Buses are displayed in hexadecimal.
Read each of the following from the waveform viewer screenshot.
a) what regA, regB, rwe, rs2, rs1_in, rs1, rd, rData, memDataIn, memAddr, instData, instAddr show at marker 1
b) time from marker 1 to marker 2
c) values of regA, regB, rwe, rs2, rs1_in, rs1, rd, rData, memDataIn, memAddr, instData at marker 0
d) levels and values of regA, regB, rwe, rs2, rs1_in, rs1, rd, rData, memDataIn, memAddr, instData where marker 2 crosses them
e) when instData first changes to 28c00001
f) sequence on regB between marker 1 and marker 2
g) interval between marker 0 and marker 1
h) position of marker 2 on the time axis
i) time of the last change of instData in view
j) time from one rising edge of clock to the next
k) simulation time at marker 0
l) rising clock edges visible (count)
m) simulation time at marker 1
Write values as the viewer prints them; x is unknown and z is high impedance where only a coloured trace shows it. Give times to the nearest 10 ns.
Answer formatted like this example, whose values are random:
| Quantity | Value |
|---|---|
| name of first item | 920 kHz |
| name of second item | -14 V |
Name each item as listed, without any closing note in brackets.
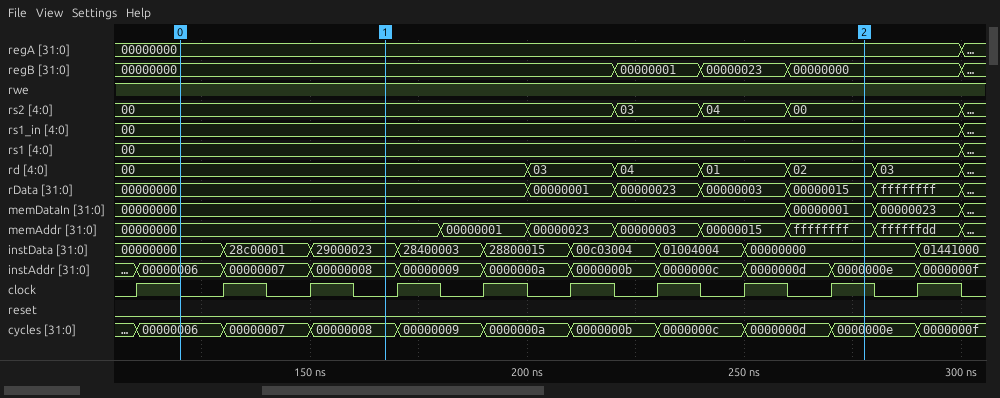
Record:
| Quantity | Value |
|---|---|
| what regA, regB, rwe, rs2, rs1_in, rs1, rd, rData, memDataIn, memAddr, instData, instAddr show at marker 1 | regA=00000000, regB=00000000, rwe=1, rs2=00, rs1_in=00, rs1=00, rd=00, rData=00000000, memDataIn=00000000, memAddr=00000000, instData=29000023, instAddr=00000008 |
| time from marker 1 to marker 2 | 110 ns |
| values of regA, regB, rwe, rs2, rs1_in, rs1, rd, rData, memDataIn, memAddr, instData at marker 0 | regA=00000000, regB=00000000, rwe=1, rs2=00, rs1_in=00, rs1=00, rd=00, rData=00000000, memDataIn=00000000, memAddr=00000000, instData=00000000 |
| levels and values of regA, regB, rwe, rs2, rs1_in, rs1, rd, rData, memDataIn, memAddr, instData where marker 2 crosses them | regA=00000000, regB=00000000, rwe=1, rs2=00, rs1_in=00, rs1=00, rd=02, rData=00000015, memDataIn=00000001, memAddr=ffffffff, instData=00000000 |
| when instData first changes to 28c00001 | 130 ns |
| sequence on regB between marker 1 and marker 2 | 00000000, 00000001, 00000023, 00000000 |
| interval between marker 0 and marker 1 | 50 ns |
| position of marker 2 on the time axis | 280 ns |
| time of the last change of instData in view | 290 ns |
| time from one rising edge of clock to the next | 20 ns |
| simulation time at marker 0 | 120 ns |
| rising clock edges visible | 10 |
| simulation time at marker 1 | 170 ns |
